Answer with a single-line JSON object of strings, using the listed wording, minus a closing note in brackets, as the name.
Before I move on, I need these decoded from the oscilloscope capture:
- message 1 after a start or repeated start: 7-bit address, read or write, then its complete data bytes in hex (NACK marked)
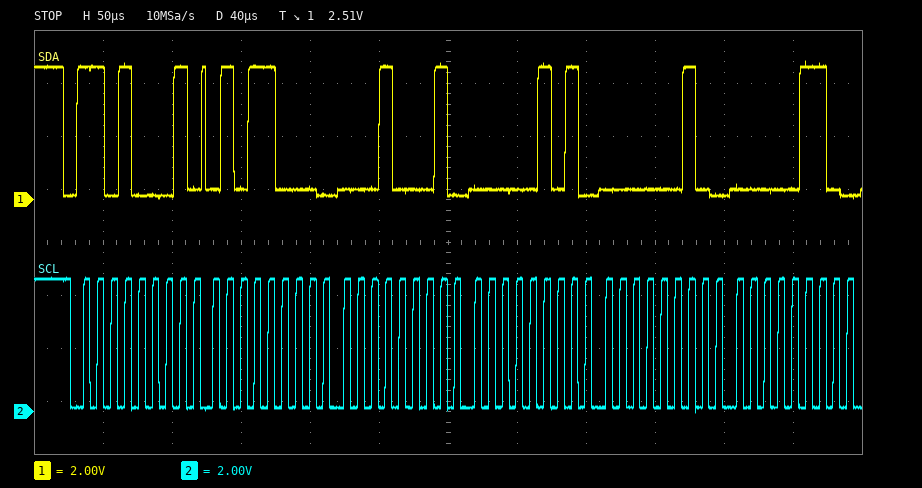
{"message 1 after a start or repeated start: 7-bit address, read or write, then its complete data bytes in hex": "0x68 read: 58 11 05 02 06"}
